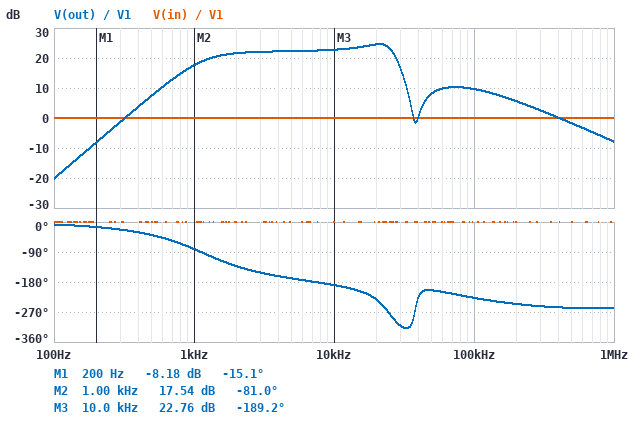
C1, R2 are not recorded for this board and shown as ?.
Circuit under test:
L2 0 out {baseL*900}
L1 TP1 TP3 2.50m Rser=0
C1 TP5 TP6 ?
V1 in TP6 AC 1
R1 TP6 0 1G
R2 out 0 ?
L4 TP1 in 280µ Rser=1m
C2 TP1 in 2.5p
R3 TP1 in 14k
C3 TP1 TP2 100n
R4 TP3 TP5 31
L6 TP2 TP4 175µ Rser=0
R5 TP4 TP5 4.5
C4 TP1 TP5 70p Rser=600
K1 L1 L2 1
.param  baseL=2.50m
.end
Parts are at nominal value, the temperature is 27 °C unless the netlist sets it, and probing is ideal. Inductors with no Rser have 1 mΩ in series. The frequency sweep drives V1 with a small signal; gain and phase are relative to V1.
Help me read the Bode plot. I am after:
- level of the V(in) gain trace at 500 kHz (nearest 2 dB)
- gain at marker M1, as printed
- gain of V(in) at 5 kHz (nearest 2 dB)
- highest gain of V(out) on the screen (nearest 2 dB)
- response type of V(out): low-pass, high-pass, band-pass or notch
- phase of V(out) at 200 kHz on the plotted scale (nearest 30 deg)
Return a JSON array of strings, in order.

["0 dB", "-8.18 dB", "0 dB", "24 dB", "band-pass", "-240 deg"]
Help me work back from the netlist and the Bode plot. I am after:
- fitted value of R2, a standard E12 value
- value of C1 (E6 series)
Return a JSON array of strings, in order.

["22 kΩ", "3.3 µF"]
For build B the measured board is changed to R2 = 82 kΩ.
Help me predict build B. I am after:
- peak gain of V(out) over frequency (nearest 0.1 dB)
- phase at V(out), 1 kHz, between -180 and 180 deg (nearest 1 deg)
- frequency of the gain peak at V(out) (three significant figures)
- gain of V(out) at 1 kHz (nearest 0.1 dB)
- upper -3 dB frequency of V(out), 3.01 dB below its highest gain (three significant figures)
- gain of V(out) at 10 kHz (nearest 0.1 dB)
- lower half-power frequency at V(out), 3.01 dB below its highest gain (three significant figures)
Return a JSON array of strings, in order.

["34.0 dB", "-58 deg", "23.5 kHz", "20.0 dB", "26.2 kHz", "27.2 dB", "19.1 kHz"]
